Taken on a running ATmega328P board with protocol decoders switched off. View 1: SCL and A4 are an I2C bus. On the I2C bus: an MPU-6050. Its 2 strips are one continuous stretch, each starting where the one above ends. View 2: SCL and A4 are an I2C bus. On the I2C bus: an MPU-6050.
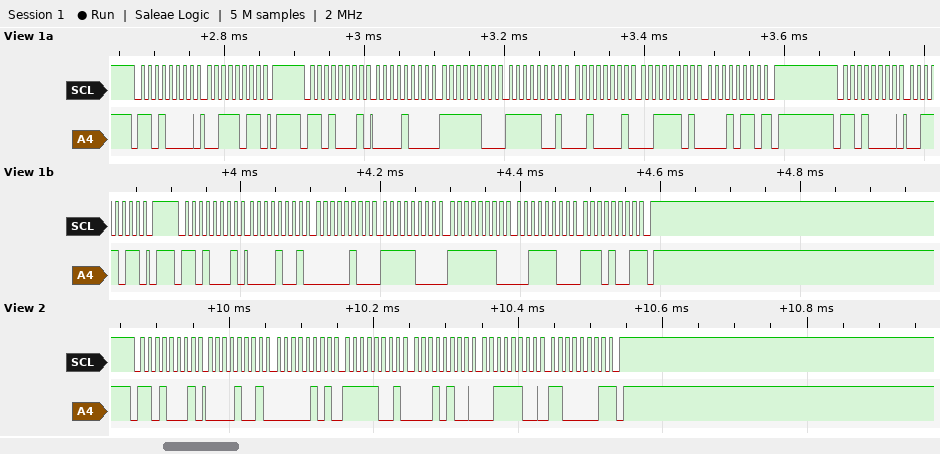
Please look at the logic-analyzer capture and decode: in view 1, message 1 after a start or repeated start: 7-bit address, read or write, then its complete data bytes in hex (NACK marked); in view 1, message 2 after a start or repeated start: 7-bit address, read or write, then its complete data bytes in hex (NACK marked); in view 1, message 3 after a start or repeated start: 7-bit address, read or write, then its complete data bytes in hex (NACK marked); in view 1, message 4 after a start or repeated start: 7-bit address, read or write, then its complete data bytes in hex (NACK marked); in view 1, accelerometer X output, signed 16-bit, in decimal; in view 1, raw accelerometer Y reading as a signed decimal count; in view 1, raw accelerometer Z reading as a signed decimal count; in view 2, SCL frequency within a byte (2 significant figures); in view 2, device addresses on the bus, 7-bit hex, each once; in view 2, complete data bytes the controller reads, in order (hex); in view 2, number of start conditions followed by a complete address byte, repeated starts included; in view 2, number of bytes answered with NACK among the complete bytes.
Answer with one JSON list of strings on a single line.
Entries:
["0x68 write: 3B", "0x68 read: 08 FC F9 21 3D 16 NACK", "0x68 write: 3B", "0x68 read: 09 04 F8 FE 3C E9 NACK", "2300", "-1759", "15638", "100 kHz", "0x68", "09 05 F9 14 3C C1", "1", "1"]
